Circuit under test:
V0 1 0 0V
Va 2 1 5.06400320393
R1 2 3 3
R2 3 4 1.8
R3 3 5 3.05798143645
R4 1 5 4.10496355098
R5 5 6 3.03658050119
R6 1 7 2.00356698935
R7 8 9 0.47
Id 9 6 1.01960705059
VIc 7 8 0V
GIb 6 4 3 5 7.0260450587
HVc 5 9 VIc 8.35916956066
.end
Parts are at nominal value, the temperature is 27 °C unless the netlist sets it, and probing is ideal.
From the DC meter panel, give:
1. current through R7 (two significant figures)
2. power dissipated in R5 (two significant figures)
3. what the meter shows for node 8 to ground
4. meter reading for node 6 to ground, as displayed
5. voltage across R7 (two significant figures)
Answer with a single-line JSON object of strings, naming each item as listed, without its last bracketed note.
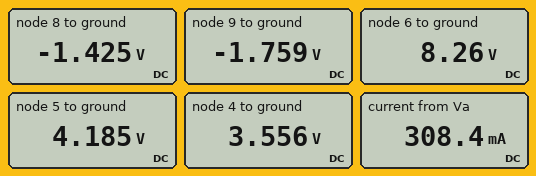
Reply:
{"current through R7": "710 mA", "power dissipated in R5": "5.5 W", "what the meter shows for node 8 to ground": "-1.425 V", "meter reading for node 6 to ground, as displayed": "8.26 V", "voltage across R7": "330 mV"}
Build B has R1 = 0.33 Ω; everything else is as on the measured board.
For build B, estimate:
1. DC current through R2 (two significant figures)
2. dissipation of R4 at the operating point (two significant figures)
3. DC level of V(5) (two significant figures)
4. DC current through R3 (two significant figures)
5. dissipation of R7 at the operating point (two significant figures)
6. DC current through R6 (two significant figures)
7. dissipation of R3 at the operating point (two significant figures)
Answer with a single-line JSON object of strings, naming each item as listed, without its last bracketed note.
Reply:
{"DC current through R2": "390 mA", "dissipation of R4 at the operating point": "6.1 W", "DC level of V(5)": "5.0 V", "DC current through R3": "18 mA", "dissipation of R7 at the operating point": "340 mW", "DC current through R6": "850 mA", "dissipation of R3 at the operating point": "990 µW"}
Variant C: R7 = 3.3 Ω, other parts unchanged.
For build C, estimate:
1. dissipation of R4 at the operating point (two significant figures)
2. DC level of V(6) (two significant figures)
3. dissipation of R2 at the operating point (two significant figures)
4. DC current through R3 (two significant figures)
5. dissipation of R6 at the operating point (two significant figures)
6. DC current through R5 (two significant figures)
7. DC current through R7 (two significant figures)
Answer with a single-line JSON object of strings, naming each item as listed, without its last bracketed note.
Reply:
{"dissipation of R4 at the operating point": "11 W", "DC level of V(6)": "8.0 V", "dissipation of R2 at the operating point": "610 mW", "DC current through R3": "27 mA", "dissipation of R6 at the operating point": "9.5 W", "DC current through R5": "440 mA", "DC current through R7": "2.2 A"}
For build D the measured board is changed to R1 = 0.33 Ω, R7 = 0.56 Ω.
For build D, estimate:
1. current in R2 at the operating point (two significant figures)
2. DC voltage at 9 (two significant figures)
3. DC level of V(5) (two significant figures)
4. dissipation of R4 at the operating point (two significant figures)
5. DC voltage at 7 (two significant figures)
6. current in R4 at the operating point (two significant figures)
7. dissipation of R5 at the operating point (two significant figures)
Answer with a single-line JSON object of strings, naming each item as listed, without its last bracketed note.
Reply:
{"current in R2 at the operating point": "370 mA", "DC voltage at 9": "-2.2 V", "DC level of V(5)": "5.0 V", "dissipation of R4 at the operating point": "6.1 W", "DC voltage at 7": "-1.7 V", "current in R4 at the operating point": "1.2 A", "dissipation of R5 at the operating point": "5.9 W"}
